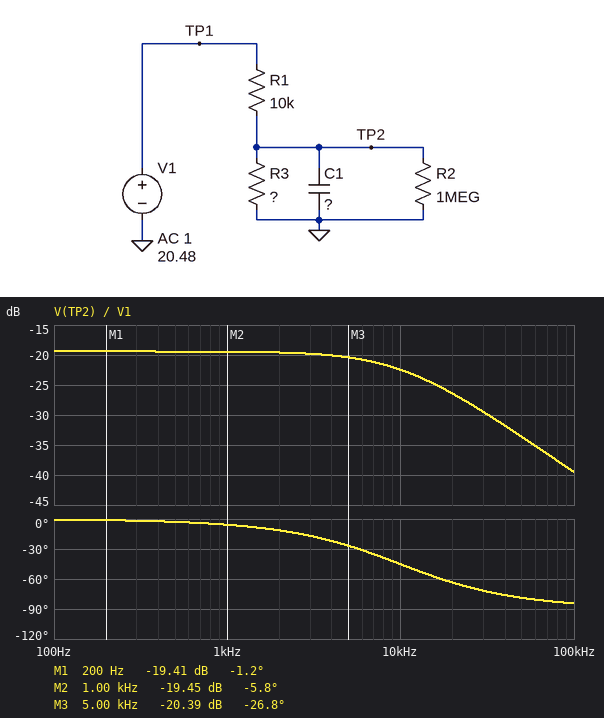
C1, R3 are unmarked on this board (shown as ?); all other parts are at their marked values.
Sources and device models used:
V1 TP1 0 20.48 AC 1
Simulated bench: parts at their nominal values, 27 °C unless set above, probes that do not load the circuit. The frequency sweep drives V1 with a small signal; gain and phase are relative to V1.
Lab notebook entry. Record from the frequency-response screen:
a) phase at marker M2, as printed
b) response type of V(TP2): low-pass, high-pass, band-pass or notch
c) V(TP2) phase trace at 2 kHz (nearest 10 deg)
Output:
-5.8 deg
low-pass
-10 deg
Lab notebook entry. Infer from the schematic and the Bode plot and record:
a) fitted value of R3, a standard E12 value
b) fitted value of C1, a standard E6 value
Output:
1.2 kΩ
15 nF
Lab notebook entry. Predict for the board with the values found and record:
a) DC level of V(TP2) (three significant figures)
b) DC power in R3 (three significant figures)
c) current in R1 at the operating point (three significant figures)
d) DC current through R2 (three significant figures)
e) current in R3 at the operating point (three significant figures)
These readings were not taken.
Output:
2.19 V
4.00 mW
1.83 mA
2.19 µA
1.83 mA
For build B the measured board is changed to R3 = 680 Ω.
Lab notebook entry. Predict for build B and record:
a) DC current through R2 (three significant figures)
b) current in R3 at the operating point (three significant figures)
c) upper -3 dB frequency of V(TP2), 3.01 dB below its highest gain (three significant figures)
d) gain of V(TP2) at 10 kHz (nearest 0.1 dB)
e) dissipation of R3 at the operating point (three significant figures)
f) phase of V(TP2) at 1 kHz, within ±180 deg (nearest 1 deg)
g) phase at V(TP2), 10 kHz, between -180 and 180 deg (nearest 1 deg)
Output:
1.30 µA
1.92 mA
16.7 kHz
-25.3 dB
2.50 mW
-3 deg
-31 deg
